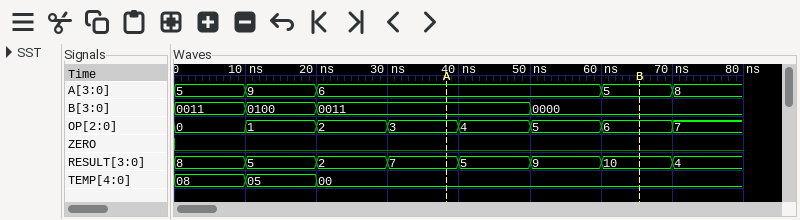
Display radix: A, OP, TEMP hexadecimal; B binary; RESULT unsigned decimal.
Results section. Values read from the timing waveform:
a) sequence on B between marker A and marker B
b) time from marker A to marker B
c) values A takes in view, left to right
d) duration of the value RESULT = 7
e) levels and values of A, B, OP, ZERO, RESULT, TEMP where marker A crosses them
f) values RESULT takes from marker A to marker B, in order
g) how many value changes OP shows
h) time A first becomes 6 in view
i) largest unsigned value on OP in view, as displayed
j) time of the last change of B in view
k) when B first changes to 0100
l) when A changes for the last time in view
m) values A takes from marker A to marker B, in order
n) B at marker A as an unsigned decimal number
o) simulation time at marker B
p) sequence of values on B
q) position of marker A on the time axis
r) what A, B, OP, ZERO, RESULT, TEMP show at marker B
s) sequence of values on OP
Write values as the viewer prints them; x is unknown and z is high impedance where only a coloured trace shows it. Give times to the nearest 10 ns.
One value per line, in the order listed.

0011, 0000
30 ns
5, 9, 6, 5, 8
10 ns
A=6, B=0011, OP=3, ZERO=0, RESULT=7, TEMP=00
7, 5, 9, 10
7
20 ns
7
50 ns
10 ns
70 ns
6, 5
3
70 ns
0011, 0100, 0011, 0000
40 ns
A=5, B=0000, OP=6, ZERO=0, RESULT=10, TEMP=00
0, 1, 2, 3, 4, 5, 6, 7
